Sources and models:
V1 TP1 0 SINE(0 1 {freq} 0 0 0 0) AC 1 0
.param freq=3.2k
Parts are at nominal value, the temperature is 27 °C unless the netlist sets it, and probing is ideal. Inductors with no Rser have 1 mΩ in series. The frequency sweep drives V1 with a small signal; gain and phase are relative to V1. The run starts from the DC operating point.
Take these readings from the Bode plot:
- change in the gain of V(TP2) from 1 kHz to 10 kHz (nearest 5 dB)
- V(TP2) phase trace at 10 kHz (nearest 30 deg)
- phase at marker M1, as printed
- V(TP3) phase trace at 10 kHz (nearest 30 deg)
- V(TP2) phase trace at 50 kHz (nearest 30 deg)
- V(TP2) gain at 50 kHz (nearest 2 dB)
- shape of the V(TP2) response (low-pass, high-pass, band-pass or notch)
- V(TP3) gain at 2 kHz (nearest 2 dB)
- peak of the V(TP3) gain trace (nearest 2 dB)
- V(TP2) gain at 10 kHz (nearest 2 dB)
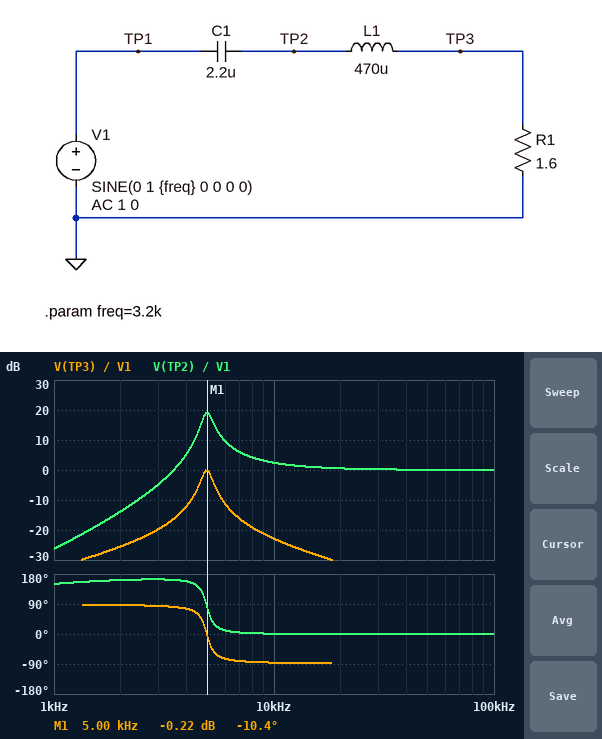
30 dB
0 deg
-10.4 deg
-90 deg
0 deg
0 dB
high-pass
-26 dB
0 dB
2 dB
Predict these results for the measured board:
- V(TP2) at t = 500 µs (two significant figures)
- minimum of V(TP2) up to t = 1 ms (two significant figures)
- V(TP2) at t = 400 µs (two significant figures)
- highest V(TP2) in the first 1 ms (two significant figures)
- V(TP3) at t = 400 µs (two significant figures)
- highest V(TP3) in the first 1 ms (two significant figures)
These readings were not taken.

410 mV
-1.2 V
-900 mV
1.4 V
-67 mV
190 mV
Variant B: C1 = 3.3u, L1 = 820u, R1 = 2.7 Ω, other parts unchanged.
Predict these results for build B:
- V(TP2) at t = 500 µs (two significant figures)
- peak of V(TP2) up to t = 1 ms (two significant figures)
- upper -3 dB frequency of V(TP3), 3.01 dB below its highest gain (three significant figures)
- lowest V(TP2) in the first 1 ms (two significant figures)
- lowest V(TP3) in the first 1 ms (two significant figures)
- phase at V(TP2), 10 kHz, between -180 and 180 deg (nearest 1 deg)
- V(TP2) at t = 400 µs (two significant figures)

-3.4 V
4.8 V
3.33 kHz
-4.5 V
-760 mV
0 deg
570 mV
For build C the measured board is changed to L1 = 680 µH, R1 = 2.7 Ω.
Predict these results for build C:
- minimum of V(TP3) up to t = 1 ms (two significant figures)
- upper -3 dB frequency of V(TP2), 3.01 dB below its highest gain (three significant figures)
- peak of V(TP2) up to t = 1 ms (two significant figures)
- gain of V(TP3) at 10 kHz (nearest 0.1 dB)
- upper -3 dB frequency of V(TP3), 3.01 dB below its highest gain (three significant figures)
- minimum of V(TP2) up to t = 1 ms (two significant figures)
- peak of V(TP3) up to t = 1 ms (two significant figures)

-390 mV
4.50 kHz
2.1 V
-22.4 dB
4.44 kHz
-2.2 V
370 mV
